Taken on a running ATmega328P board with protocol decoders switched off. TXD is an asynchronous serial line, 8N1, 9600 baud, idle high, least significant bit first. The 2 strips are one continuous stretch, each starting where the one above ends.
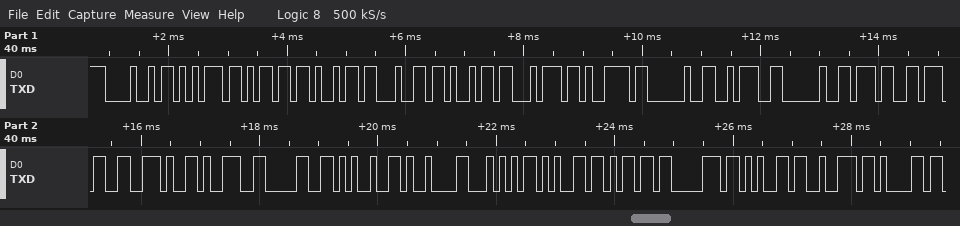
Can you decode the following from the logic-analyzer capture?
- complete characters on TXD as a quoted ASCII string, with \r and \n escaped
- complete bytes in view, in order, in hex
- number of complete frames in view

"Humidity : 77.90%\tTempera"
48 75 6D 69 64 69 74 79 20 3A 20 37 37 2E 39 30 25 09 54 65 6D 70 65 72 61
25
